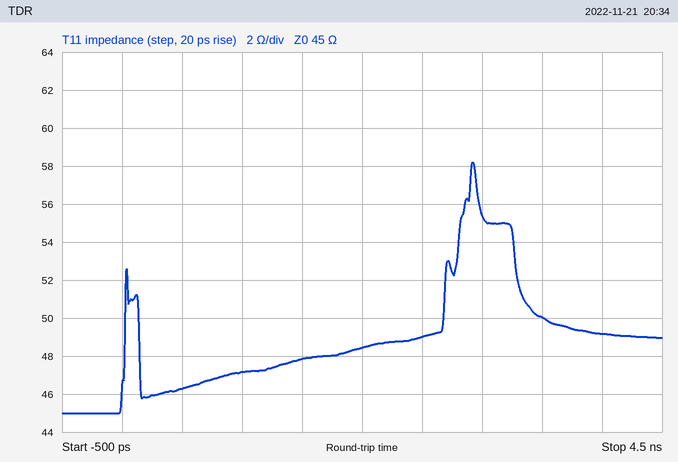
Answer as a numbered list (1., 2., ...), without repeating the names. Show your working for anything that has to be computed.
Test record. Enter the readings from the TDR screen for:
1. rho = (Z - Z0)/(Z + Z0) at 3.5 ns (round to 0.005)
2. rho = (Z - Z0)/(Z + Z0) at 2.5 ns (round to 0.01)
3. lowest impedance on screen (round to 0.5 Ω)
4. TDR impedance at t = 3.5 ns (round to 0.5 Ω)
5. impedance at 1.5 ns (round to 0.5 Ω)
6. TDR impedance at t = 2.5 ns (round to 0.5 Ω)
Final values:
1. (50 − 45)/(50 + 45) ≈ +0.0526, so +0.055 to the nearest 0.005
2. (49 − 45)/(49 + 45) ≈ +0.04
3. 45.0 Ω
4. 50.0 Ω
5. 48.0 Ω
6. 49.0 Ω
